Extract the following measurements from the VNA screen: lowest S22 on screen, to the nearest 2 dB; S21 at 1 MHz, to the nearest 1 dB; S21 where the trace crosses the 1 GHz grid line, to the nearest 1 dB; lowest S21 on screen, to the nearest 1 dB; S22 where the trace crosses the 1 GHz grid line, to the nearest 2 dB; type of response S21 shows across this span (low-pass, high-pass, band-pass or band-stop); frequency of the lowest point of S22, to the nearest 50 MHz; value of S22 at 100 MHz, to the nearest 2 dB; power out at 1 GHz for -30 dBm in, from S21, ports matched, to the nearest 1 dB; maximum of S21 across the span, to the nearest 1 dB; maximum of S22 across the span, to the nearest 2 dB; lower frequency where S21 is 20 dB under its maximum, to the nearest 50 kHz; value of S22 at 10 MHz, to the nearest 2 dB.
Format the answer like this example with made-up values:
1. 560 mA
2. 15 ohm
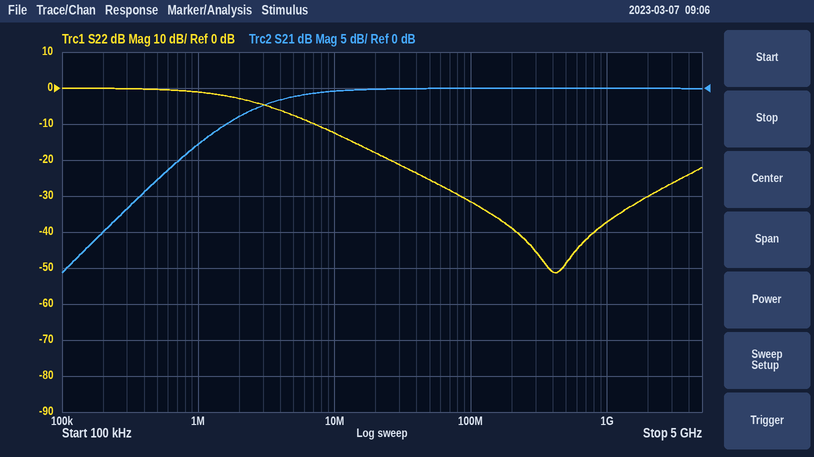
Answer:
1. -52 dB
2. -8 dB
3. 0 dB
4. -26 dB
5. -38 dB
6. high-pass
7. 400 MHz
8. -32 dB
9. -30 dBm
10. 0 dB
11. 0 dB
12. 200 kHz
13. -12 dB
